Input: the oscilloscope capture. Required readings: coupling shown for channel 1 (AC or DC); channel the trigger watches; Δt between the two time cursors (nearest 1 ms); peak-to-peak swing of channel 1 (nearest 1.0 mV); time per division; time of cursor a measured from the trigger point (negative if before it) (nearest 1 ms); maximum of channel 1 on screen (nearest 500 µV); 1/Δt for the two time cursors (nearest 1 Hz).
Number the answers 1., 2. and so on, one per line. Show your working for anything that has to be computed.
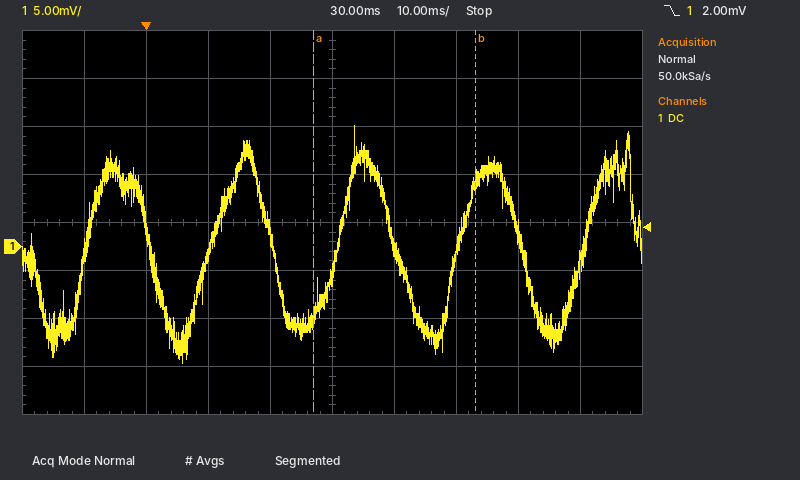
1. DC
2. channel 1
3. 26 ms
4. 25.0 mV
5. 10 ms
6. +27 ms
7. 12.5 mV
8. 1 / 26 ms ≈ 38 Hz
